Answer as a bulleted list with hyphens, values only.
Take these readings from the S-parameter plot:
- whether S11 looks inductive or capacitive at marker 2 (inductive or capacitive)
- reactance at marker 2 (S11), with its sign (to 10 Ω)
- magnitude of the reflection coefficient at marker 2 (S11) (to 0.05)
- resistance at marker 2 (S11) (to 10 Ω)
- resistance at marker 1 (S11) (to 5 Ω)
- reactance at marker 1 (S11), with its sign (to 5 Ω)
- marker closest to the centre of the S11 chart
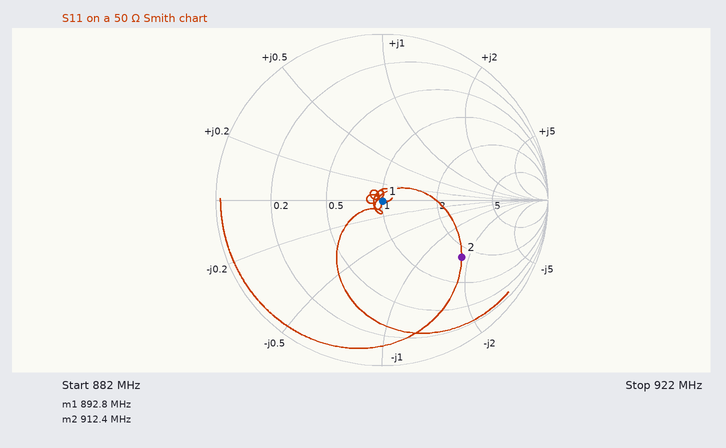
- capacitive
- -90 Ω
- 0.60
- 80 Ω
- 50 Ω
- 0 Ω
- marker 1
